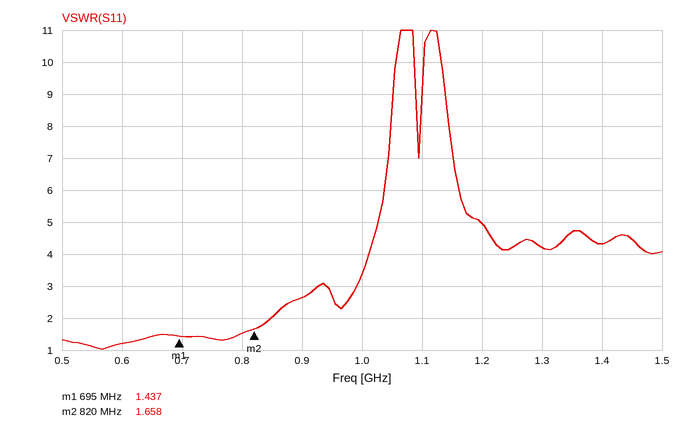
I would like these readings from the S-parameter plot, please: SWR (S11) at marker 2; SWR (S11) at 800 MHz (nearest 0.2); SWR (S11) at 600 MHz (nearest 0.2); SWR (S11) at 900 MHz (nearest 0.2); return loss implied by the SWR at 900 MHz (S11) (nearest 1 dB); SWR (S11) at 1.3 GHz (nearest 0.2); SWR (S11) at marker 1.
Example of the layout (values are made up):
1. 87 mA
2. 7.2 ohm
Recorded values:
1. 1.658
2. 1.6
3. 1.2
4. 2.6
5. 7 dB
6. 4.2
7. 1.437
